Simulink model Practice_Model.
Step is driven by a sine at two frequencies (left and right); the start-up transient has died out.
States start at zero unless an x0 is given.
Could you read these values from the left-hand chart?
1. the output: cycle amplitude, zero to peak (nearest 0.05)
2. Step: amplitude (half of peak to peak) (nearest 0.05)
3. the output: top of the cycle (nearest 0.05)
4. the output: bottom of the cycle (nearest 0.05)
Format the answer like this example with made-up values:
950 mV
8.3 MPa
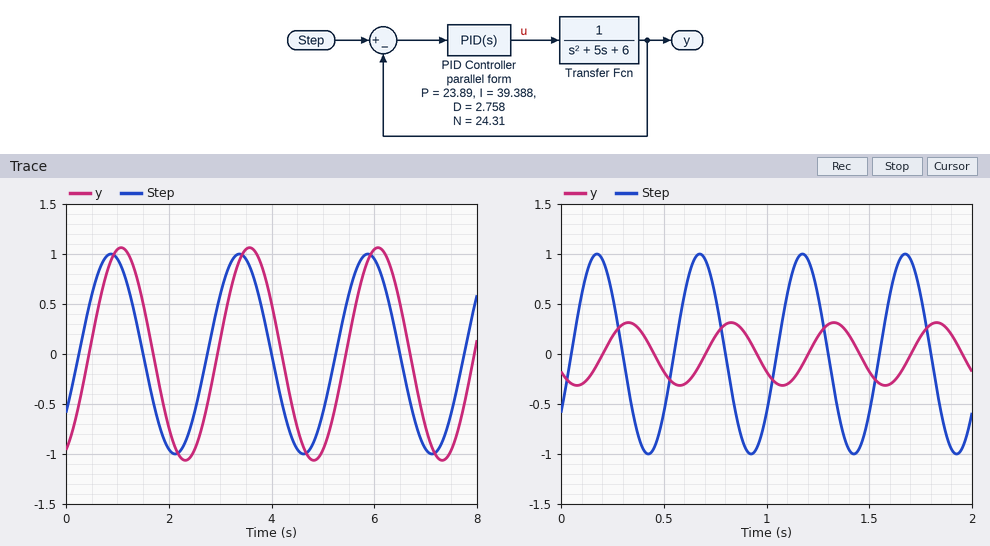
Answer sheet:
1.05
1.00
1.05
-1.05
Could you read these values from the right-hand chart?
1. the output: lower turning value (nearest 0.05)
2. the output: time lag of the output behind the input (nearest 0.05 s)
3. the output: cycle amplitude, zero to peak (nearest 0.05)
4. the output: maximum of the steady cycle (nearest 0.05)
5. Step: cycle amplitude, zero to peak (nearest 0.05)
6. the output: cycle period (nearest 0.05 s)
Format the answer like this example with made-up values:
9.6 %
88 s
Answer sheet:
-0.30
0.15 s
0.30
0.30
1.00
0.50 s
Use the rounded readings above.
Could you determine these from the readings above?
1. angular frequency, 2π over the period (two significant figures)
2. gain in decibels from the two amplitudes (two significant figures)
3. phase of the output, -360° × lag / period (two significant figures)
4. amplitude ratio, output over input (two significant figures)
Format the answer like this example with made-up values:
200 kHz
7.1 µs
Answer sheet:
13 rad/s
-10 dB
-110°
0.30
